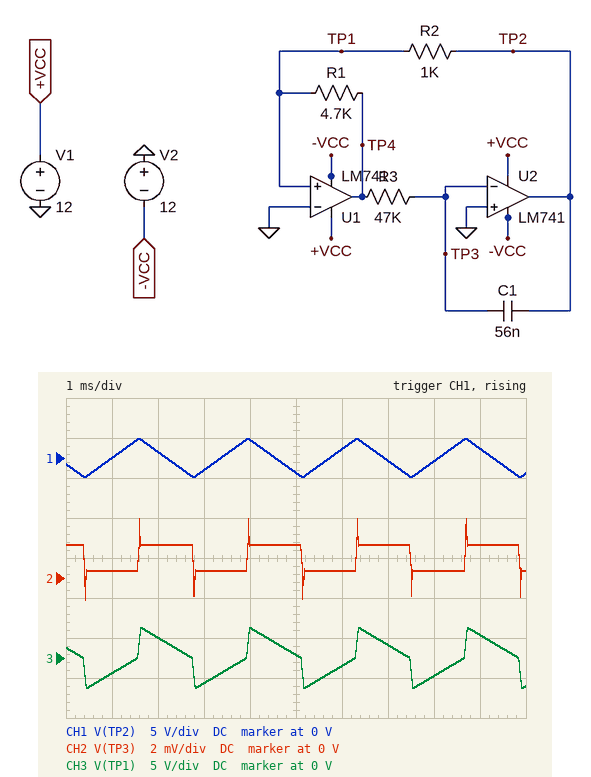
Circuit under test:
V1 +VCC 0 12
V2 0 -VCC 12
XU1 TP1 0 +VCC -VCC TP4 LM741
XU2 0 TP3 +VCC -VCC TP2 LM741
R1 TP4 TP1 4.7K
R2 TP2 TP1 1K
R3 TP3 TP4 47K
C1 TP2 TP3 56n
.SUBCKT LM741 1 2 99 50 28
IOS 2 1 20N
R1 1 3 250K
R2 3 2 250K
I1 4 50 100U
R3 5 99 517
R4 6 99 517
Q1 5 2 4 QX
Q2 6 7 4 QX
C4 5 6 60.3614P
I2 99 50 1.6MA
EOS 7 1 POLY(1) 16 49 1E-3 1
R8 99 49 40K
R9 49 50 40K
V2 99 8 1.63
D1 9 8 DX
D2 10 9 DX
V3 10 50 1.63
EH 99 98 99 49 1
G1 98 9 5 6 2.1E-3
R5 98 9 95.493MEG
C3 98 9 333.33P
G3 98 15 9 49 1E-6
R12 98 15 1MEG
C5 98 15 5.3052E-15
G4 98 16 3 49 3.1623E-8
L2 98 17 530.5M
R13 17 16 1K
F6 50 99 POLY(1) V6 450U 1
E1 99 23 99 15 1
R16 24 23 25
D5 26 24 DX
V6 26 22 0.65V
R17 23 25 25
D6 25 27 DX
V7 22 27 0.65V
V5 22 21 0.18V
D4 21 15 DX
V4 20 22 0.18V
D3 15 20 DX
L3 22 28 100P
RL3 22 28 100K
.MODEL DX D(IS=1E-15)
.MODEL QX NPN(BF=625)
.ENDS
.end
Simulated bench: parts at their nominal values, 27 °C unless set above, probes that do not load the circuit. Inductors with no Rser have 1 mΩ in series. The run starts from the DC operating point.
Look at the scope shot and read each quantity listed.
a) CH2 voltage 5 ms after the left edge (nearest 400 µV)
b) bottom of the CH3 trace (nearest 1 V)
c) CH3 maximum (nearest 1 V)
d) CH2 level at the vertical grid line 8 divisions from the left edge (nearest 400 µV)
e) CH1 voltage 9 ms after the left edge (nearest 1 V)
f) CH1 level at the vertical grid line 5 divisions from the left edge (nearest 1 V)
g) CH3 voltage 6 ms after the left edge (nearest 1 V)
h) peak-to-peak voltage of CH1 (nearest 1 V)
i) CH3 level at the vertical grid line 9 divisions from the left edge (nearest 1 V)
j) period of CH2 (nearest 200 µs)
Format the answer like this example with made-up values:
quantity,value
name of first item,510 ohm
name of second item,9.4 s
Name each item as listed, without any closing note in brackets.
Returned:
quantity,value
CH2 voltage 5 ms after the left edge,1.6 mV
bottom of the CH3 trace,-4 V
CH3 maximum,4 V
CH2 level at the vertical grid line 8 divisions from the left edge,400 µV
CH1 voltage 9 ms after the left edge,1 V
CH1 level at the vertical grid line 5 divisions from the left edge,-2 V
CH3 voltage 6 ms after the left edge,-1 V
peak-to-peak voltage of CH1,5 V
CH3 level at the vertical grid line 9 divisions from the left edge,3 V
period of CH2,2.4 ms
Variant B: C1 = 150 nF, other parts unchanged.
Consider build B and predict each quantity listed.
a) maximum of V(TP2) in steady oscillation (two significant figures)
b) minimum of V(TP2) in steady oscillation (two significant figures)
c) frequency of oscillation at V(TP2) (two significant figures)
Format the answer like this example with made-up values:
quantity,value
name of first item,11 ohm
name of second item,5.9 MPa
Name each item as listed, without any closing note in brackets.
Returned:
quantity,value
maximum of V(TP2) in steady oscillation,2.3 V
minimum of V(TP2) in steady oscillation,-2.3 V
frequency of oscillation at V(TP2),160 Hz
